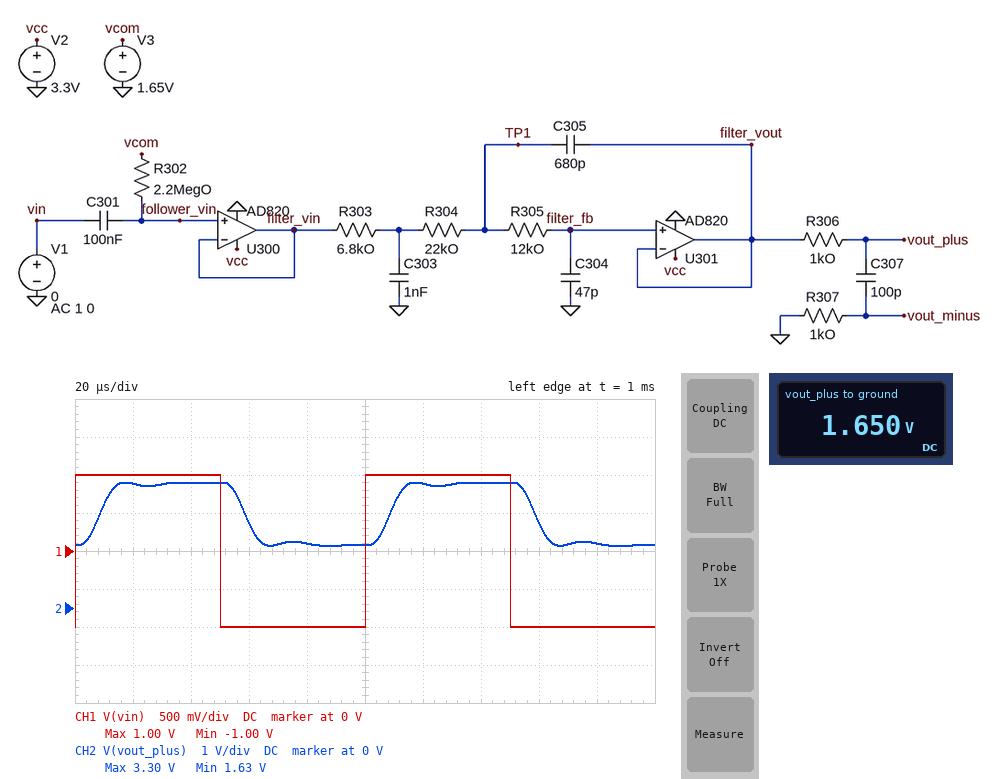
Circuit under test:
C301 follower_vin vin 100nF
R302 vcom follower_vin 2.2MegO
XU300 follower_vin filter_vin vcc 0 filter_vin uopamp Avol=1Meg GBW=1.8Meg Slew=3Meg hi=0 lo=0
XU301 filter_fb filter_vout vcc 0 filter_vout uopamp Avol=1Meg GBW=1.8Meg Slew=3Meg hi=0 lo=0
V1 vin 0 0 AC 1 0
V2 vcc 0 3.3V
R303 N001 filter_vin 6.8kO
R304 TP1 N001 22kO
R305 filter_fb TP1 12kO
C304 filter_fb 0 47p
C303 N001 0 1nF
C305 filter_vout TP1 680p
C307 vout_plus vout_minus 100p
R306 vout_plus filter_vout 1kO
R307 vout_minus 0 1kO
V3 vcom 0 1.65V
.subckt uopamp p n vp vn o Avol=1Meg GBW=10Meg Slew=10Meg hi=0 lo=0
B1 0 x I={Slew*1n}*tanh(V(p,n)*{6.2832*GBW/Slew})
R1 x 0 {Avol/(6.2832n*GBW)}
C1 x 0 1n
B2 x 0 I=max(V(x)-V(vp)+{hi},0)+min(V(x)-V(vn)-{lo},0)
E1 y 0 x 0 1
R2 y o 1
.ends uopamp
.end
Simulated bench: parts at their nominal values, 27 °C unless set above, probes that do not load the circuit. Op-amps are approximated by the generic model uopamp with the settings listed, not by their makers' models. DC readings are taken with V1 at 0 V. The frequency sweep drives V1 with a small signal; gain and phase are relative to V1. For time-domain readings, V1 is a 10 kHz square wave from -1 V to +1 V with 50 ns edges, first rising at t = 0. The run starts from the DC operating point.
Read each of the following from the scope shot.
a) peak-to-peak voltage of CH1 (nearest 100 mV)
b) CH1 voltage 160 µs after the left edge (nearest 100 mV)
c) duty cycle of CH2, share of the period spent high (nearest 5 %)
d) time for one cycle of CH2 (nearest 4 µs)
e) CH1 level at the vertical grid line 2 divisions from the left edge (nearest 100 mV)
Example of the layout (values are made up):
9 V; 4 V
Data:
2.0 V; -1.0 V; 50 %; 100 µs; 1.0 V
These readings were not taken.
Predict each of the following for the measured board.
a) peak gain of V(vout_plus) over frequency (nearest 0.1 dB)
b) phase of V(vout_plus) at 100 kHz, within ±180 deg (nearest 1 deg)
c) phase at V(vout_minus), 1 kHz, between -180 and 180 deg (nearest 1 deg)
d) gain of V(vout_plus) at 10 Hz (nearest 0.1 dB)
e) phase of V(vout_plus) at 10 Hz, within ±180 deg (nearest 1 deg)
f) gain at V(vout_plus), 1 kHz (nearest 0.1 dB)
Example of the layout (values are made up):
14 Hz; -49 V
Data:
0 dB; 118 deg; 87 deg; 0 dB; 4 deg; 0 dB
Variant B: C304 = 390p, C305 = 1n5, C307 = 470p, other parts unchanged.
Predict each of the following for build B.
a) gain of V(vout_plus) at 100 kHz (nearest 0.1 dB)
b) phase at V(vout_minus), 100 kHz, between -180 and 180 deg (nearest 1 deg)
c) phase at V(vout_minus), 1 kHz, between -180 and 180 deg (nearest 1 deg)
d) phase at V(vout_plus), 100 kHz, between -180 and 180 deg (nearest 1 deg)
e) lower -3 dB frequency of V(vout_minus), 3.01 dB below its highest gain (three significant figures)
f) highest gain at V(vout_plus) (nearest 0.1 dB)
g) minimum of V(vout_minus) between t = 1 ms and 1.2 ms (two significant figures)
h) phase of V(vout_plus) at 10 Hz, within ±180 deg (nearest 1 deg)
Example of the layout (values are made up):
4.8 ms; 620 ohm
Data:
-49.8 dB; 168 deg; 81 deg; 94 deg; 5.97 kHz; 0.2 dB; -26 mV; 4 deg
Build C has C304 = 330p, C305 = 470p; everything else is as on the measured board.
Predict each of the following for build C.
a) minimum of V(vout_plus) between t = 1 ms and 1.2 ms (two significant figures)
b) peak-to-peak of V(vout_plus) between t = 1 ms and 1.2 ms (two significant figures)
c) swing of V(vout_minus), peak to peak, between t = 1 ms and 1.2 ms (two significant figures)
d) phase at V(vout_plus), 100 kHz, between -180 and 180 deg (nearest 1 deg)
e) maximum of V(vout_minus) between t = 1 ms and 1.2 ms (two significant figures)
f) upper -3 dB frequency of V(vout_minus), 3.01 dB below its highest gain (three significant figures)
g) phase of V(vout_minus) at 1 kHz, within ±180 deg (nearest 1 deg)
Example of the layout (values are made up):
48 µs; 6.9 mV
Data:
1.7 V; 1.6 V; 13 mV; 121 deg; 6.6 mV; 34.7 kHz; 83 deg
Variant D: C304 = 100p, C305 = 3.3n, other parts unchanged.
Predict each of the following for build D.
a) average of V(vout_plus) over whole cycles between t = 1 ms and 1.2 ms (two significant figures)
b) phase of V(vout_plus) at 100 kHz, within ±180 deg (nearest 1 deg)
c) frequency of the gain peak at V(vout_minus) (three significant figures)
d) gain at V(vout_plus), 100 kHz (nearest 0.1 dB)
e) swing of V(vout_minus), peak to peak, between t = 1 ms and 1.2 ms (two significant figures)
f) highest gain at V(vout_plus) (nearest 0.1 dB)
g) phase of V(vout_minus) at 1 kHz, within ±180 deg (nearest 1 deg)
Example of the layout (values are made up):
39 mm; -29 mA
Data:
2.4 V; 101 deg; 14.6 kHz; -44.2 dB; 24 mV; 5.4 dB; 86 deg
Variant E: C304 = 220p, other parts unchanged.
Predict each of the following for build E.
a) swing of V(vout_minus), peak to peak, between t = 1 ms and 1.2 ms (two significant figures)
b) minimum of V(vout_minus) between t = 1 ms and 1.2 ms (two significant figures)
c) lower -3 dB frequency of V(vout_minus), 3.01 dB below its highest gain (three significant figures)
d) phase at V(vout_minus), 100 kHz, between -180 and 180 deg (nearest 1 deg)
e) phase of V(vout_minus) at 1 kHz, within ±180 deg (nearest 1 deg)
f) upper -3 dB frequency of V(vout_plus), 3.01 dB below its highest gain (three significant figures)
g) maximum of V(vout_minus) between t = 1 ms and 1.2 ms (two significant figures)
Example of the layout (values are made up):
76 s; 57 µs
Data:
17 mV; -8.6 mV; 9.81 kHz; -159 deg; 84 deg; 17.9 kHz; 8.5 mV
